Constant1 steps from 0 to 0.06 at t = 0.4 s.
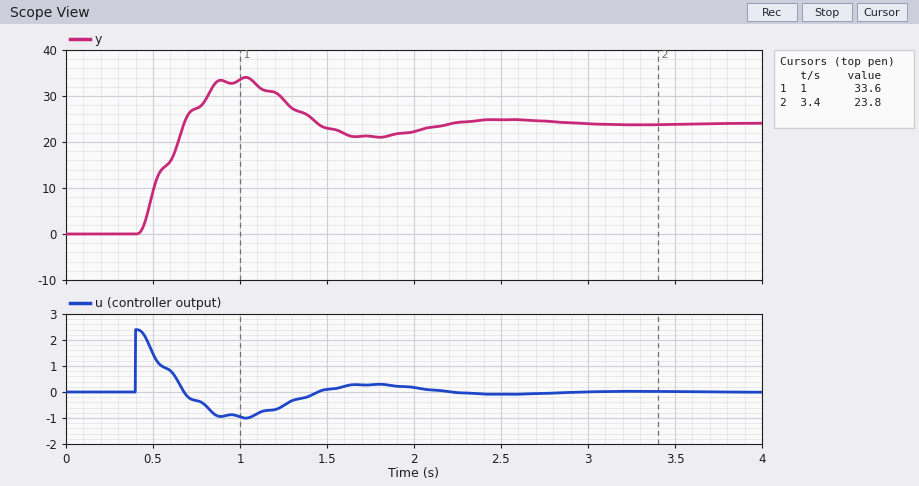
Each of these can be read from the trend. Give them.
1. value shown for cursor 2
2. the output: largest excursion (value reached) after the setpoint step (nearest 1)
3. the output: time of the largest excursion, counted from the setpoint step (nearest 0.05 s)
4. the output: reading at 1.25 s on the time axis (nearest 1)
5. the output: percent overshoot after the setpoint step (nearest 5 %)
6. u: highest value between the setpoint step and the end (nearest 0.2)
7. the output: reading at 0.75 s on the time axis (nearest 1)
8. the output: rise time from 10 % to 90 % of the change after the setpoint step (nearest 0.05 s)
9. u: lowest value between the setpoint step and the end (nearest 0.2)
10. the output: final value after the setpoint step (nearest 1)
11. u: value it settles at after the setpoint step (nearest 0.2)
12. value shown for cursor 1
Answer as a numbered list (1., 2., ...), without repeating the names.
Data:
1. 23.8
2. 34
3. 0.65 s
4. 29
5. 40 %
6. 2.4
7. 27
8. 0.20 s
9. -1.0
10. 24
11. 0.0
12. 33.6
